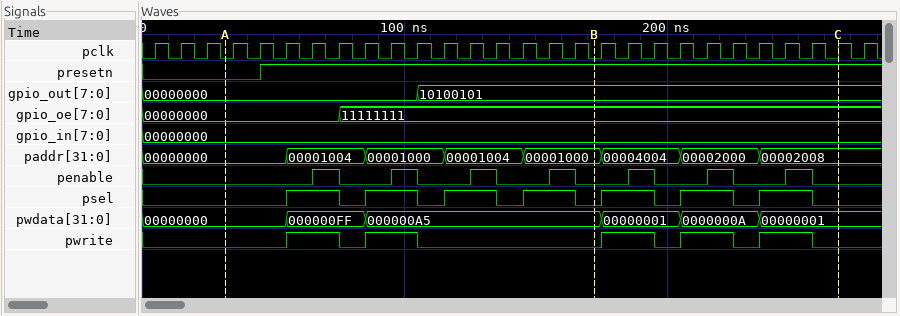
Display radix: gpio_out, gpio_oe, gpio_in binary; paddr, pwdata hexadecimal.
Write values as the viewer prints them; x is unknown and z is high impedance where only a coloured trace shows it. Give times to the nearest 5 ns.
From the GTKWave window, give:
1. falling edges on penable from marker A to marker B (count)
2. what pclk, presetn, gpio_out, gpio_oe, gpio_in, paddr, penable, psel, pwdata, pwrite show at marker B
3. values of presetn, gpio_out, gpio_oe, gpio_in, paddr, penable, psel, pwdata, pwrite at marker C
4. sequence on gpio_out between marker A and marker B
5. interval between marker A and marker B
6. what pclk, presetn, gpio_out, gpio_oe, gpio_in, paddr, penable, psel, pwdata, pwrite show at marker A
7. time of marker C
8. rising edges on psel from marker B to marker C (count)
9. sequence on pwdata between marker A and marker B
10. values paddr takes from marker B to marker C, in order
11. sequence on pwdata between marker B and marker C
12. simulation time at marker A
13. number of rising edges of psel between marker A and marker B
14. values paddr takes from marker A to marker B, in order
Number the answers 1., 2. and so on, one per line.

1. 4
2. pclk=0, presetn=1, gpio_out=10100101, gpio_oe=11111111, gpio_in=00000000, paddr=00001000, penable=0, psel=0, pwdata=000000A5, pwrite=0
3. presetn=1, gpio_out=10100101, gpio_oe=11111111, gpio_in=00000000, paddr=00002008, penable=0, psel=0, pwdata=00000001, pwrite=0
4. 00000000, 10100101
5. 140 ns
6. pclk=0, presetn=0, gpio_out=00000000, gpio_oe=00000000, gpio_in=00000000, paddr=00000000, penable=0, psel=0, pwdata=00000000, pwrite=0
7. 265 ns
8. 3
9. 00000000, 000000FF, 000000A5
10. 00001000, 00004004, 00002000, 00002008
11. 000000A5, 00000001, 0000000A, 00000001
12. 30 ns
13. 4
14. 00000000, 00001004, 00001000, 00001004, 00001000
